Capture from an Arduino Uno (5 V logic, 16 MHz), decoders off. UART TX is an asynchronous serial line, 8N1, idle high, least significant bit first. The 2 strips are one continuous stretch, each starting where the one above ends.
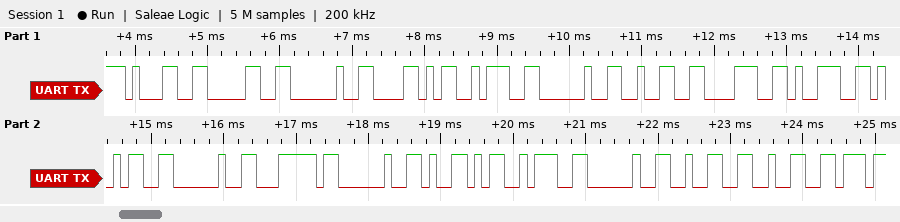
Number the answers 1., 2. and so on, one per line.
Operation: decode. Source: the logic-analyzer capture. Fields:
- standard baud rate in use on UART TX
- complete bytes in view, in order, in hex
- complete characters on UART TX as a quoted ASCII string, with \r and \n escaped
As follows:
1. 9600 baud
2. 31 30 20 58 3A 20 32 38 39 35 20 7C 20 59 3A 20 32 32
3. "10 X: 2895 | Y: 22"
